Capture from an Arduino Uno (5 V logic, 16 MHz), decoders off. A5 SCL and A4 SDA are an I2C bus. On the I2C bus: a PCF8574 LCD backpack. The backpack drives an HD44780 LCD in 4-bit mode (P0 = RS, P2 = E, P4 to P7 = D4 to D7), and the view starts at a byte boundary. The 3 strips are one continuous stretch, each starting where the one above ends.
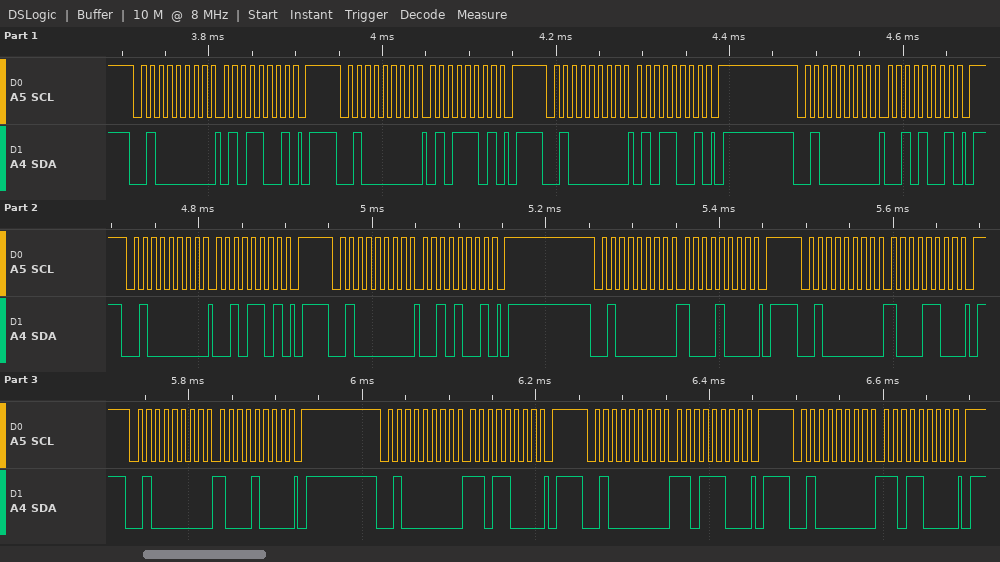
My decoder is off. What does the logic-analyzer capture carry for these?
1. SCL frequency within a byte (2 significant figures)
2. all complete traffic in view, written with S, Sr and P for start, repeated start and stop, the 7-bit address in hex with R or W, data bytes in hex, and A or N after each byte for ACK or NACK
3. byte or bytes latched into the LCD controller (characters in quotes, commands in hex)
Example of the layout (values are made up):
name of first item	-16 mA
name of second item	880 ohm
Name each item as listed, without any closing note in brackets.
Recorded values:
SCL frequency within a byte	100 kHz
all complete traffic in view, written with S, Sr and P for start, repeated start and stop, the 7-bit address in hex with R or W, data bytes in hex, and A or N after each byte for ACK or NACK	S 20W A 59 A P S 20W A 5D A P S 20W A 59 A P S 20W A 29 A P S 20W A 2D A P S 20W A 29 A P S 20W A 88 A P S 20W A 8C A P S 20W A 88 A P S 20W A D8 A P S 20W A DC A P S 20W A D8 A P
byte or bytes latched into the LCD controller	'R' 0x8D
